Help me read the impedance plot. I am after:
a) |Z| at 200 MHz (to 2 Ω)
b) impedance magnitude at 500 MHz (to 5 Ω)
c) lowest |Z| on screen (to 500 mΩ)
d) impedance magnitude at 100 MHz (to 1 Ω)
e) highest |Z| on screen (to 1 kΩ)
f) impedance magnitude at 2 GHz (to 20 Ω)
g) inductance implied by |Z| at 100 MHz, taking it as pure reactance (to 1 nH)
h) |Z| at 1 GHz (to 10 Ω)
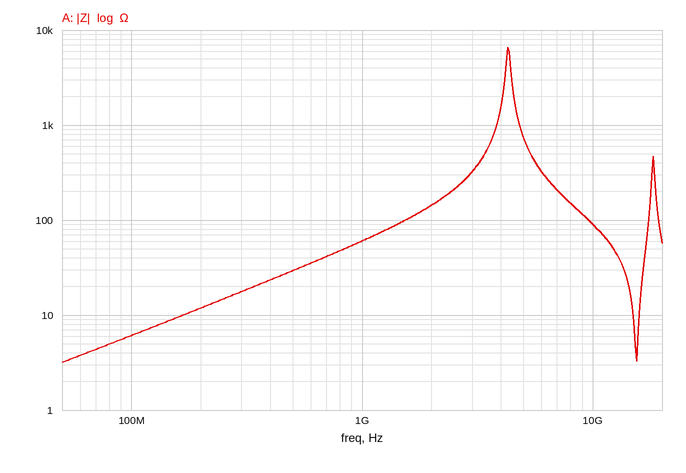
12 Ω
30 Ω
3.0 Ω
6 Ω
7 kΩ
140 Ω
10 nH
60 Ω
